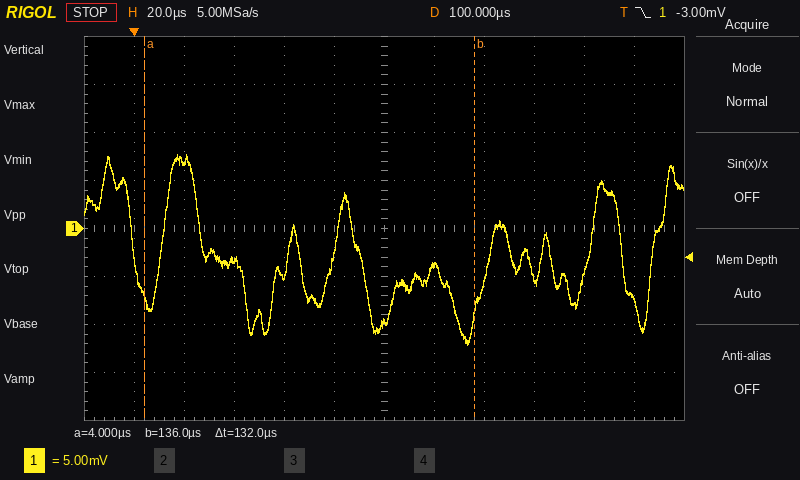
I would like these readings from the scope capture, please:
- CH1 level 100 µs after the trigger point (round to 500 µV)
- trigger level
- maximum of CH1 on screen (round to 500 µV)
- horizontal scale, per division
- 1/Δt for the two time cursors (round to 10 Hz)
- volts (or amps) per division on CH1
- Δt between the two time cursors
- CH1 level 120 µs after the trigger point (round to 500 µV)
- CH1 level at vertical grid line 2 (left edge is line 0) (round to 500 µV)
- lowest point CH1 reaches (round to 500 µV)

-10.0 mV
-3.00 mV
7.5 mV
20 µs
7.58 kHz
5 mV
132 µs
-4.0 mV
7.0 mV
-12.0 mV
